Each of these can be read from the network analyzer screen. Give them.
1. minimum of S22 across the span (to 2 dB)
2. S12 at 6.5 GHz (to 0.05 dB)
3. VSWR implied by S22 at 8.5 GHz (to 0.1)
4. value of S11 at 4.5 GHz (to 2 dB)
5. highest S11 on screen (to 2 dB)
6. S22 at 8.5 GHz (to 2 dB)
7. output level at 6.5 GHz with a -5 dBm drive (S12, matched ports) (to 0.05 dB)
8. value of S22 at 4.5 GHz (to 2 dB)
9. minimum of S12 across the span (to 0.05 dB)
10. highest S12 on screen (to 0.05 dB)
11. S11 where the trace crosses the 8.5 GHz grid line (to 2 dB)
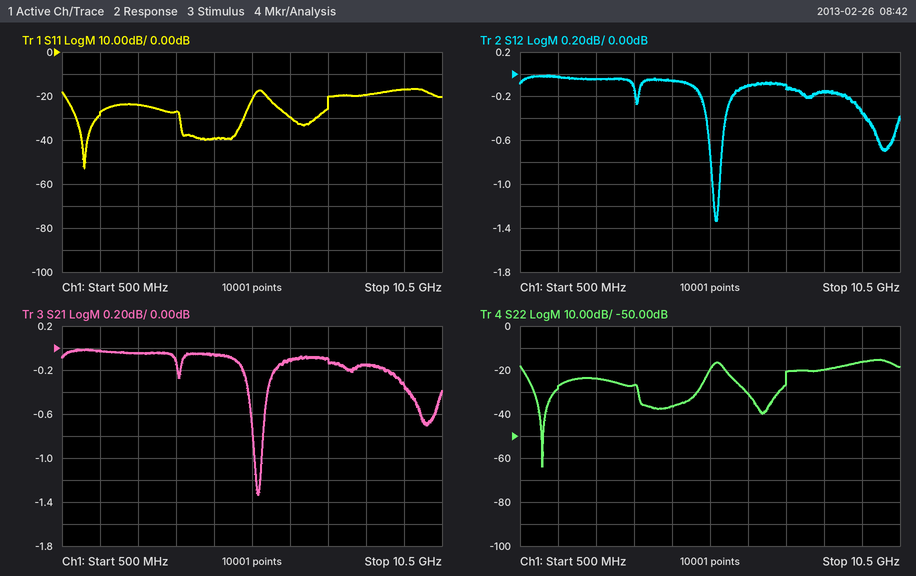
-64 dB
-0.10 dB
1.2
-40 dB
-16 dB
-20 dB
-5.10 dBm
-36 dB
-1.35 dB
0.00 dB
-20 dB
